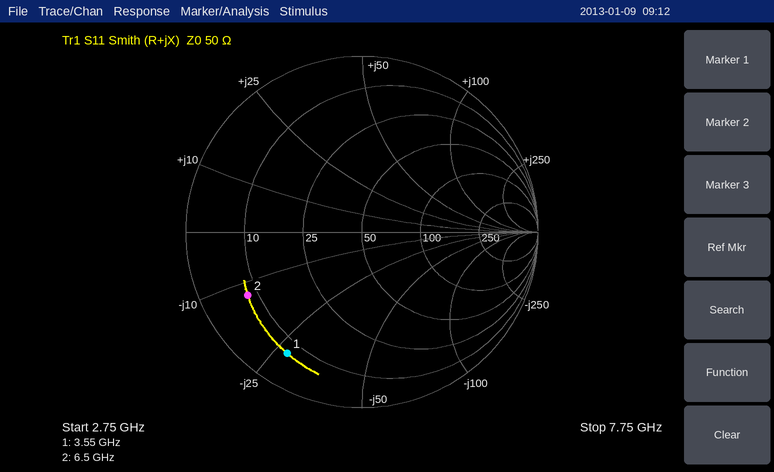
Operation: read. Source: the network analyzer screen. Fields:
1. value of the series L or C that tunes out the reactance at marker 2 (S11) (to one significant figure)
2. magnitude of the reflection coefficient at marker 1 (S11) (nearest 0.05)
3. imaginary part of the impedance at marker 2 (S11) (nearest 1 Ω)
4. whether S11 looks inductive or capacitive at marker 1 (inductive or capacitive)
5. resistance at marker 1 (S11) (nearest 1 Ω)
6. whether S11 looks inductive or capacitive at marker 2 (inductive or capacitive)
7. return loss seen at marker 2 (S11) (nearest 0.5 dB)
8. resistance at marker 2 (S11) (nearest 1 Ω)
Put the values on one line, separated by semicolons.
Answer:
300 pH; 0.80; -13 Ω; capacitive; 7 Ω; capacitive; 2.5 dB; 8 Ω
